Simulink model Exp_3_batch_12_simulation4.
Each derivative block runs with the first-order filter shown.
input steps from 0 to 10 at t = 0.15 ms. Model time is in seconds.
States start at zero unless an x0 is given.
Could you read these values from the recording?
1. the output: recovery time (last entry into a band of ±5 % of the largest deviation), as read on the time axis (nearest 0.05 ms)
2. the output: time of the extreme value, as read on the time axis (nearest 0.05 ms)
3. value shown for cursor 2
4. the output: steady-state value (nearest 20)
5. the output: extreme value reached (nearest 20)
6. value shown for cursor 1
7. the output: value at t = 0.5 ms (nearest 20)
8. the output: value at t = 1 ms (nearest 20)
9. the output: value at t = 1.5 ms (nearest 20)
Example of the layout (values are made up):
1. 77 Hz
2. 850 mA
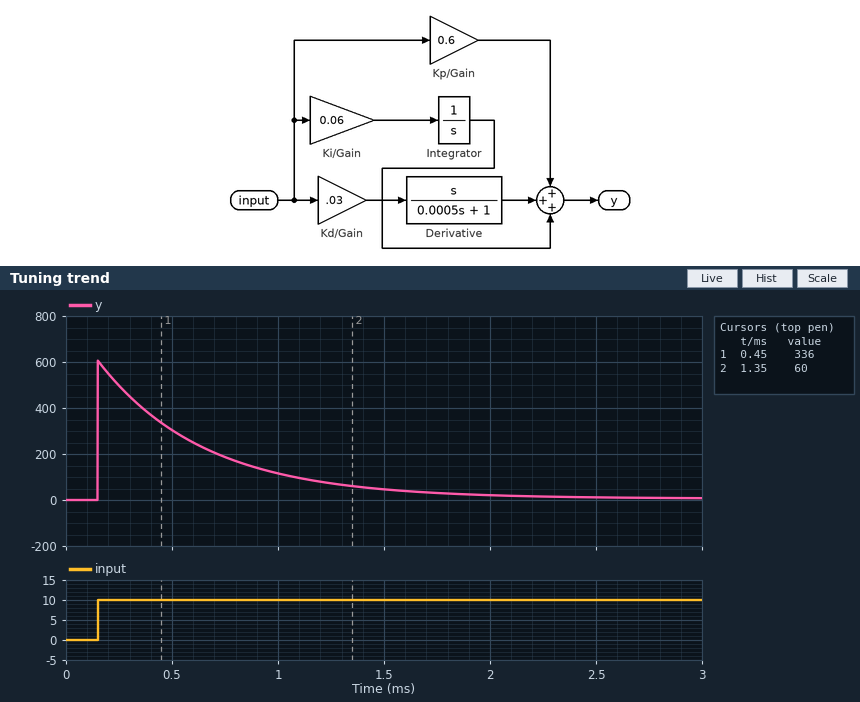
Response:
1. 1.65 ms
2. 0.15 ms
3. 60
4. 0
5. 600
6. 336
7. 300
8. 120
9. 40
